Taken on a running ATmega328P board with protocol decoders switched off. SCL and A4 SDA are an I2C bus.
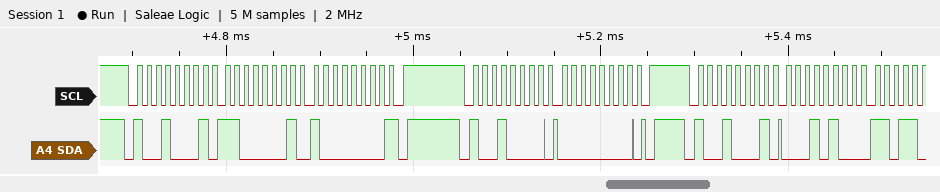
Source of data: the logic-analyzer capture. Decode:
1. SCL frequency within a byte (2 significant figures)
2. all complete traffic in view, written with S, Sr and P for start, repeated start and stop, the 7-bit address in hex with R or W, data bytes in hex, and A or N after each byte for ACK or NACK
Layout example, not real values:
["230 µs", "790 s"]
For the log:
["100 kHz", "S 48R A C1 A 80 N P S 48W A 00 A P S 48R A 14 A"]
